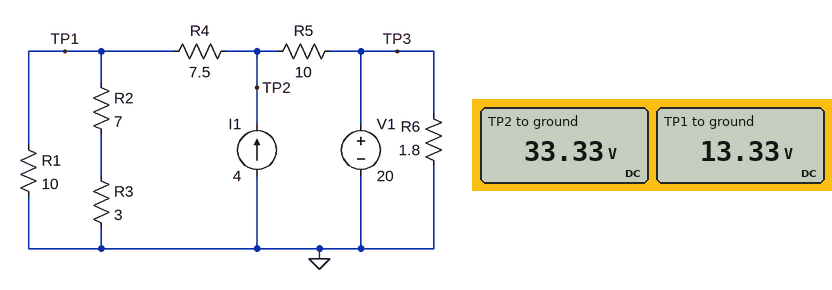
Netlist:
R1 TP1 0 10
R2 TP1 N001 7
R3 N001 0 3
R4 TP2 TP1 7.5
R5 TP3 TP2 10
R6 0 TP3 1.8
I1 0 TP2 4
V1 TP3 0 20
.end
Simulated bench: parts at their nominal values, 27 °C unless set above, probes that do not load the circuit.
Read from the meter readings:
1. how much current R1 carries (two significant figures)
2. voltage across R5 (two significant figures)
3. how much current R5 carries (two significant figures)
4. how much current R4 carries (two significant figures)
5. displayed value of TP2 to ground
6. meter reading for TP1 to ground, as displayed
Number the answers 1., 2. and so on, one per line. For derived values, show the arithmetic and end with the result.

1. (13.33 V) / 10 Ω = 1.3 A
2. 33.33 V - 20 V = 13 V
3. (33.33 V - 20 V) / 10 Ω = 1.3 A
4. (33.33 V - 13.33 V) / 7.5 Ω = 2.7 A
5. 33.33 V
6. 13.33 V
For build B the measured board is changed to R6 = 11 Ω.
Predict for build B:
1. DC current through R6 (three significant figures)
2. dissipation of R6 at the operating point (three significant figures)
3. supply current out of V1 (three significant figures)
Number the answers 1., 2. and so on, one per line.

1. 1.82 A
2. 36.4 W
3. 485 mA
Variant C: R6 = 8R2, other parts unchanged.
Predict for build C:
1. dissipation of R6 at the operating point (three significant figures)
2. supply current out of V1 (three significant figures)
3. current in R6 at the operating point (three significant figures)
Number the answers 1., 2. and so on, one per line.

1. 48.8 W
2. 1.11 A
3. 2.44 A
